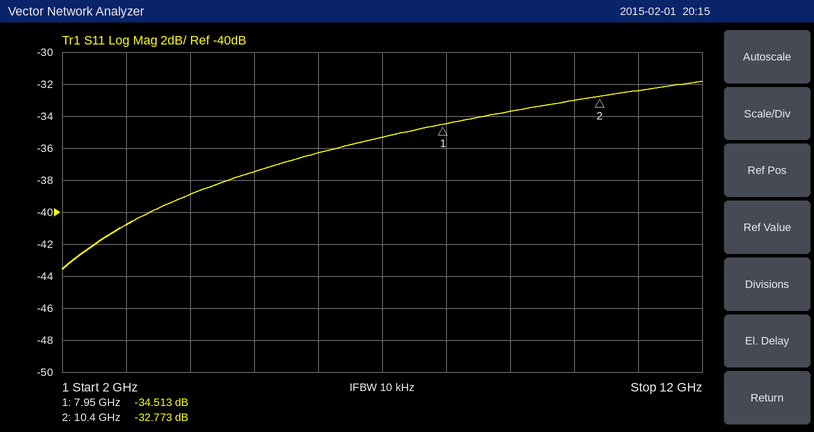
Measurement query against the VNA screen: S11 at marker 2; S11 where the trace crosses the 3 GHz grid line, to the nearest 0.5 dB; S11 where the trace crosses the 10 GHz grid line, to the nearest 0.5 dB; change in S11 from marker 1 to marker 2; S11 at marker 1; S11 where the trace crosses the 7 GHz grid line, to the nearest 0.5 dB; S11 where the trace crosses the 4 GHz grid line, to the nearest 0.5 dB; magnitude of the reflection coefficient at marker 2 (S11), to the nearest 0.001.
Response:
-32.773 dB
-41.0 dB
-33.0 dB
1.740 dB
-34.513 dB
-35.5 dB
-39.0 dB
0.023
